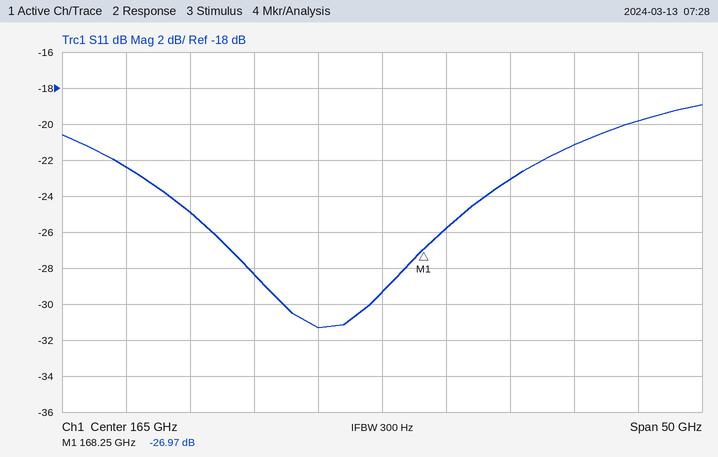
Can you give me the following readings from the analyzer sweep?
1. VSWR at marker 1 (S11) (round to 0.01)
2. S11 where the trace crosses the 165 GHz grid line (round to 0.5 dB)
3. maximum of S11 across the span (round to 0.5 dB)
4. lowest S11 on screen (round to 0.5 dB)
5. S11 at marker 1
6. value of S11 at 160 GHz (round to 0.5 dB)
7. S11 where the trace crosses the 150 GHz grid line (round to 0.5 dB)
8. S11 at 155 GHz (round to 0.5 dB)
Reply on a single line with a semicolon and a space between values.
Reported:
1.09; -29.5 dB; -19.0 dB; -31.5 dB; -26.97 dB; -31.5 dB; -25.0 dB; -28.5 dB
